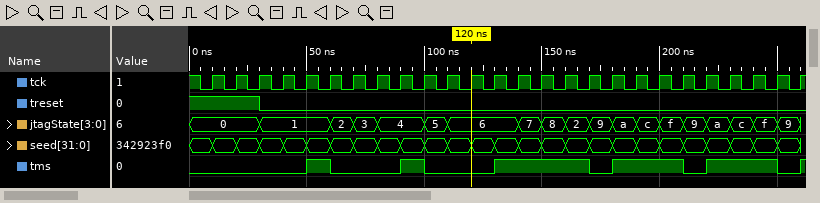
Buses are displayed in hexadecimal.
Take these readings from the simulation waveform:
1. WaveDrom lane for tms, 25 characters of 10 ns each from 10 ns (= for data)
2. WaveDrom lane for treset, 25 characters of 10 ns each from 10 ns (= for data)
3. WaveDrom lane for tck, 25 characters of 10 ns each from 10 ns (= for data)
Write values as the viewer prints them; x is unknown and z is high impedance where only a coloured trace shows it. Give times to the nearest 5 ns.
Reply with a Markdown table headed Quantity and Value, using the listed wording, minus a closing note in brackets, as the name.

| Quantity | Value |
|---|---|
| WaveDrom lane for tms, 25 characters of 10 ns each from 10 ns | {name: 'tms', wave: '0...10..10..1...01..01..0'} |
| WaveDrom lane for treset, 25 characters of 10 ns each from 10 ns | {name: 'treset', wave: '1.0......................'} |
| WaveDrom lane for tck, 25 characters of 10 ns each from 10 ns | {name: 'tck', wave: 'p........................'} |
